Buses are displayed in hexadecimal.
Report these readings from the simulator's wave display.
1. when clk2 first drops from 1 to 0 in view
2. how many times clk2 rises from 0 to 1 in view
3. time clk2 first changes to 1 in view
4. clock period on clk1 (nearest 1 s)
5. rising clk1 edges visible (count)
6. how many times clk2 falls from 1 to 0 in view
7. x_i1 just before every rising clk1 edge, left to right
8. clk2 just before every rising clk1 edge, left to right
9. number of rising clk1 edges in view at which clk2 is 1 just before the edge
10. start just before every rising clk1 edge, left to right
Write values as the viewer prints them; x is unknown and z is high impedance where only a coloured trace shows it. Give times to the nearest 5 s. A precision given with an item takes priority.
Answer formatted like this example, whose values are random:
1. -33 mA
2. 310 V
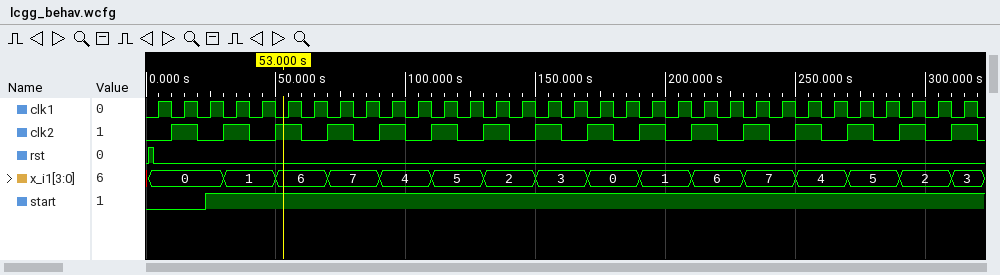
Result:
1. 20 s
2. 16
3. 10 s
4. 10 s
5. 32
6. 16
7. 0, 0, 0, 1, 1, 6, 6, 7, 7, 4, 4, 5, 5, 2, 2, 3, 3, 0, 0, 1, 1, 6, 6, 7, 7, 4, 4, 5, 5, 2, 2, 3
8. 0 1 0 1 0 1 0 1 0 1 0 1 0 1 0 1 0 1 0 1 0 1 0 1 0 1 0 1 0 1 0 1
9. 16
10. 0 0 1 1 1 1 1 1 1 1 1 1 1 1 1 1 1 1 1 1 1 1 1 1 1 1 1 1 1 1 1 1
